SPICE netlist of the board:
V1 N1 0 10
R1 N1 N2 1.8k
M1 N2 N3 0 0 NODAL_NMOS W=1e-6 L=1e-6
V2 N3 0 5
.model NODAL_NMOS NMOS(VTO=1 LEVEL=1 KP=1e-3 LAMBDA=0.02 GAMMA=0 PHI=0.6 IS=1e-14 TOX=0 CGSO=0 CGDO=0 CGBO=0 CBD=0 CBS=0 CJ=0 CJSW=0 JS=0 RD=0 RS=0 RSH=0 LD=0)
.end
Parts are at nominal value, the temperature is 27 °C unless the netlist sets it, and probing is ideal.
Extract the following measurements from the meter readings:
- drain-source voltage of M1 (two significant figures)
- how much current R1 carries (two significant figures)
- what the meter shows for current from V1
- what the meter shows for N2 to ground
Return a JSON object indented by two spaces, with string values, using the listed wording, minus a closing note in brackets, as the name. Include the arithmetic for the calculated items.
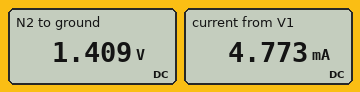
{
  "drain-source voltage of M1": "1.409 V = 1.4 V",
  "how much current R1 carries": "(10 V - 1.409 V) / 1.8 kΩ = 4.8 mA",
  "what the meter shows for current from V1": "4.773 mA",
  "what the meter shows for N2 to ground": "1.409 V"
}
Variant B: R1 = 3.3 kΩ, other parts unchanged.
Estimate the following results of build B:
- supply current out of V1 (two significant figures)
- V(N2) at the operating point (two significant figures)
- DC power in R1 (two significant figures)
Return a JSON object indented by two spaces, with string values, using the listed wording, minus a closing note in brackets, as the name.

{
  "supply current out of V1": "2.8 mA",
  "V(N2) at the operating point": "760 mV",
  "DC power in R1": "26 mW"
}
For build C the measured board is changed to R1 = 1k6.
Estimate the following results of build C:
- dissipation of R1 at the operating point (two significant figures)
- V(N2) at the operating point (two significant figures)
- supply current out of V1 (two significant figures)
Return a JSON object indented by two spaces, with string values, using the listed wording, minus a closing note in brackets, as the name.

{
  "dissipation of R1 at the operating point": "44 mW",
  "V(N2) at the operating point": "1.6 V",
  "supply current out of V1": "5.3 mA"
}
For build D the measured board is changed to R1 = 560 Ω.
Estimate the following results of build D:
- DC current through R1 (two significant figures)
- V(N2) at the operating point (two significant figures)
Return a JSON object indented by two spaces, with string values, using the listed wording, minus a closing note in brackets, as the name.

{
  "DC current through R1": "8.8 mA",
  "V(N2) at the operating point": "5.1 V"
}
